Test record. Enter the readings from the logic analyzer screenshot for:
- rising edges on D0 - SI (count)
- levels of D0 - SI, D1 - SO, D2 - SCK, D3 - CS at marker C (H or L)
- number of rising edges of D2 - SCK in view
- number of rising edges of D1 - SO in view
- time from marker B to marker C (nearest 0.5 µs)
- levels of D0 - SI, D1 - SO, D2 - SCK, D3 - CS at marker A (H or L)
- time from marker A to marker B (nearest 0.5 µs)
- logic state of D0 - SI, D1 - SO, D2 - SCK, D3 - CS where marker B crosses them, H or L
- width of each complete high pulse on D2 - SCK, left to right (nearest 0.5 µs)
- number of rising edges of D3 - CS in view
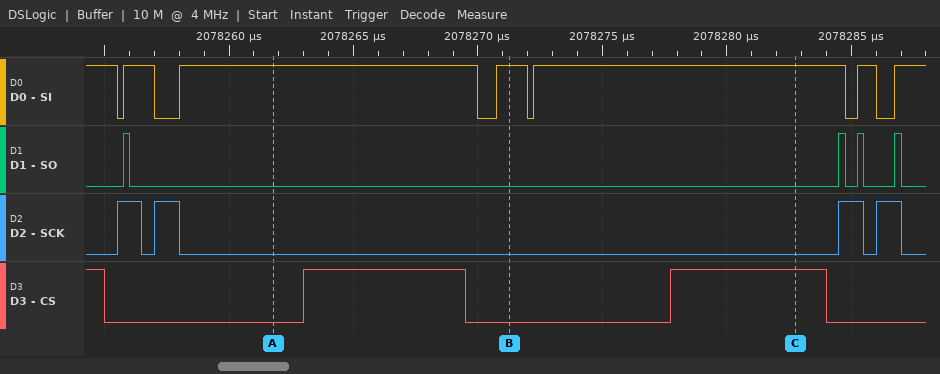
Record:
6
D0 - SI=H, D1 - SO=L, D2 - SCK=L, D3 - CS=H
4
4
11.5 µs
D0 - SI=H, D1 - SO=L, D2 - SCK=L, D3 - CS=L
9.5 µs
D0 - SI=H, D1 - SO=L, D2 - SCK=L, D3 - CS=L
1 µs, 1 µs, 1 µs, 1 µs
2
